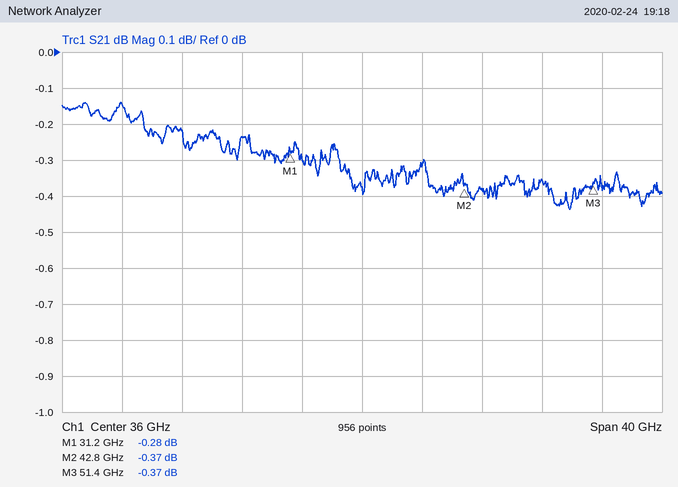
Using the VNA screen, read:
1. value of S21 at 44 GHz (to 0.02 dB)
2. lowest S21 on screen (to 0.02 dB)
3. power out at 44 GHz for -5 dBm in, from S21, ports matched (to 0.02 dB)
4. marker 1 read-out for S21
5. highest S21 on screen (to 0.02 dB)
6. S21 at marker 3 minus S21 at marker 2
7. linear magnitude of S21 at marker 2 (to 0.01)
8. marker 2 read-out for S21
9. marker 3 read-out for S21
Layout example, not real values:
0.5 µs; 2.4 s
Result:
-0.38 dB; -0.44 dB; -5.38 dBm; -0.28 dB; -0.14 dB; 0.00 dB; 0.96; -0.37 dB; -0.37 dB
